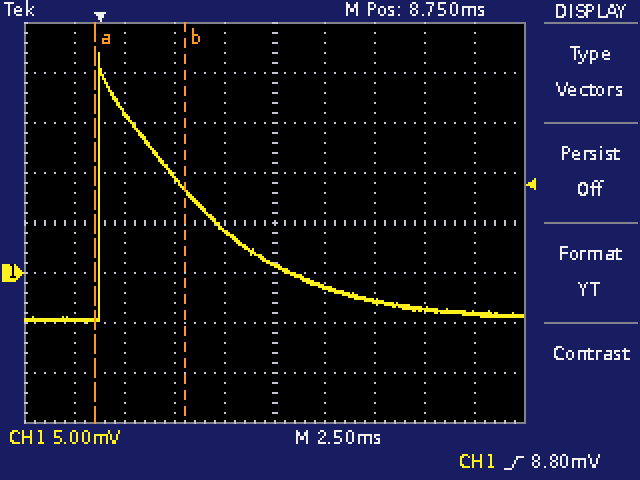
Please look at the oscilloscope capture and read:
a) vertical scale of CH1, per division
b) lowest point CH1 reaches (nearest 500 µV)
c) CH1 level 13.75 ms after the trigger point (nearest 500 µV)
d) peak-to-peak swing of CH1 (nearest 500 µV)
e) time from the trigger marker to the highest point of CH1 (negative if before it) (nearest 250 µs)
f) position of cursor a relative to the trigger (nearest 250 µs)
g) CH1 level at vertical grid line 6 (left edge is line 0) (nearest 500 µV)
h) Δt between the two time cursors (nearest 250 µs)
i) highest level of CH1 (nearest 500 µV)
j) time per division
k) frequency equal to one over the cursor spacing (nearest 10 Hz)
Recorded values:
5 mV
-5.0 mV
-3.0 mV
27.0 mV
0.00 ms
-250 µs
-1.5 mV
4.50 ms
22.0 mV
2.5 ms
220 Hz
